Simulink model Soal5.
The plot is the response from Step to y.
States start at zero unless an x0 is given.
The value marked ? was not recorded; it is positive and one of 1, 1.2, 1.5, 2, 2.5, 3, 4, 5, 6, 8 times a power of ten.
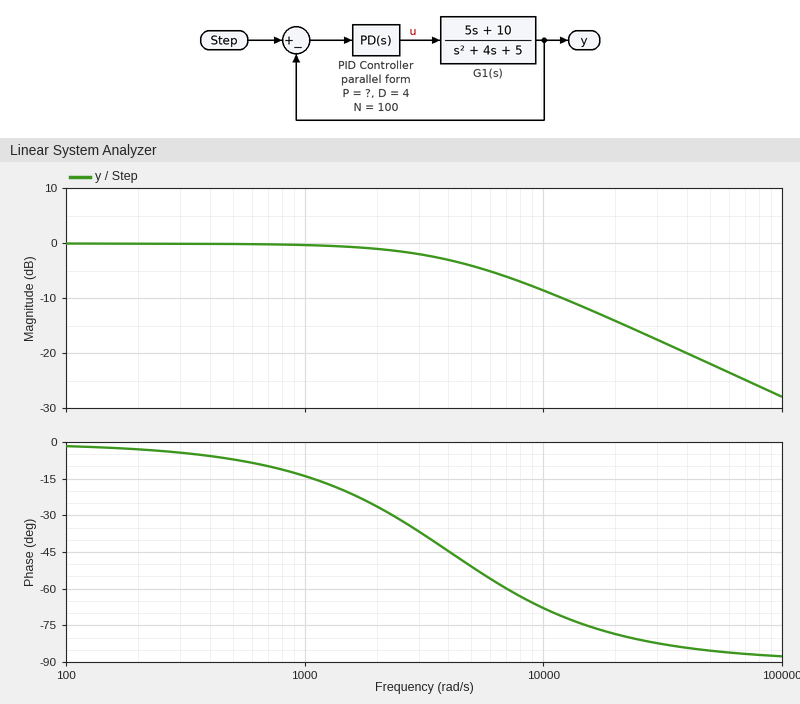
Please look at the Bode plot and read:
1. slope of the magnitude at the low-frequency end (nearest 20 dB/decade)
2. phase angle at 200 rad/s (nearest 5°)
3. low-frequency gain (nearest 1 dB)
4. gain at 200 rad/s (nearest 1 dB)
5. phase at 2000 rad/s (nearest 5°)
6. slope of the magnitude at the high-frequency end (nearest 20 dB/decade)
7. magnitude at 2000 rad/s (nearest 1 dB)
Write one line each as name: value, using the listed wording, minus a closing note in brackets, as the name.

slope of the magnitude at the low-frequency end: 0 dB/decade
phase angle at 200 rad/s: -5°
low-frequency gain: 0 dB
gain at 200 rad/s: 0 dB
phase at 2000 rad/s: -25°
slope of the magnitude at the high-frequency end: -20 dB/decade
magnitude at 2000 rad/s: -1 dB
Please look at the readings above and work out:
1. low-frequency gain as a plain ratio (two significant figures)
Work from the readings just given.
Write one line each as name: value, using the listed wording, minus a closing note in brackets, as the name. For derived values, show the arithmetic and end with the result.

low-frequency gain as a plain ratio: 10^(0 / 20) = 1.0
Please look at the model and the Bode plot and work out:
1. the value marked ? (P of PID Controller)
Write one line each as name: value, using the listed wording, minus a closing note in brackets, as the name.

the value marked ?: 400
